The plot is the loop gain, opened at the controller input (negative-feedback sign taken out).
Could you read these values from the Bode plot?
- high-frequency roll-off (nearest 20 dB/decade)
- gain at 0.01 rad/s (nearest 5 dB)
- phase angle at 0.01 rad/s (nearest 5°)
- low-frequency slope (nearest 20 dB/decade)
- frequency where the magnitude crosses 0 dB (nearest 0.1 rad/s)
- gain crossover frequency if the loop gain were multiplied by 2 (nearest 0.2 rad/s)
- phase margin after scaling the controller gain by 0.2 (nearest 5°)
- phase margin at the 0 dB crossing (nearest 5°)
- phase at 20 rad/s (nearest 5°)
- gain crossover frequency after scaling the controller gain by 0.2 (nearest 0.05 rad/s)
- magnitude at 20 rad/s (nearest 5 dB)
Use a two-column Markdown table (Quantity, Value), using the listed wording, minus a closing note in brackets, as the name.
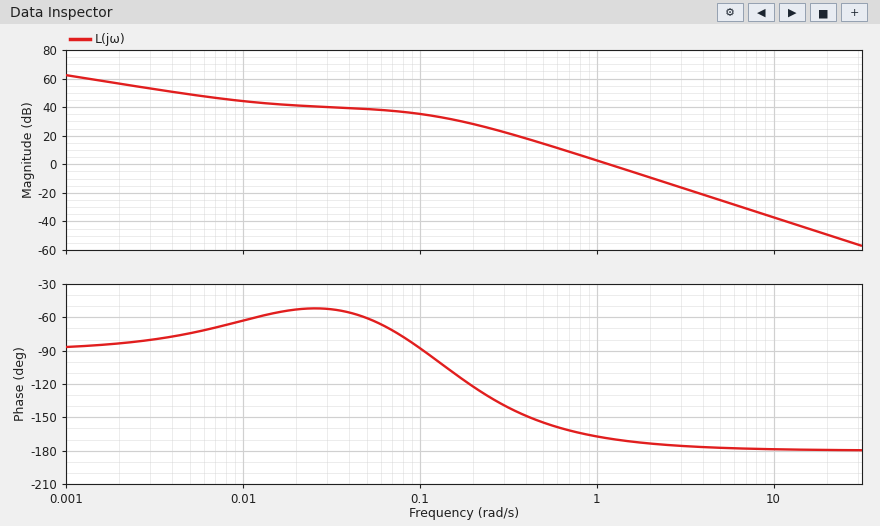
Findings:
| Quantity | Value |
|---|---|
| high-frequency roll-off | -40 dB/decade |
| gain at 0.01 rad/s | 45 dB |
| phase angle at 0.01 rad/s | -65° |
| low-frequency slope | -20 dB/decade |
| frequency where the magnitude crosses 0 dB | 1.2 rad/s |
| gain crossover frequency if the loop gain were multiplied by 2 | 1.6 rad/s |
| phase margin after scaling the controller gain by 0.2 | 25° |
| phase margin at the 0 dB crossing | 10° |
| phase at 20 rad/s | -180° |
| gain crossover frequency after scaling the controller gain by 0.2 | 0.50 rad/s |
| magnitude at 20 rad/s | -50 dB |
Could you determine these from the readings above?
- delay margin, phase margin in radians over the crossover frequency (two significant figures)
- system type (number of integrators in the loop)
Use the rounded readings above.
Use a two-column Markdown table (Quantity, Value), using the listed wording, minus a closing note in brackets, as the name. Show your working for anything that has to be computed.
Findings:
| Quantity | Value |
|---|---|
| delay margin, phase margin in radians over the crossover frequency | 10 × π / 180 / 1.2 = 0.15 s |
| system type | 1 |
